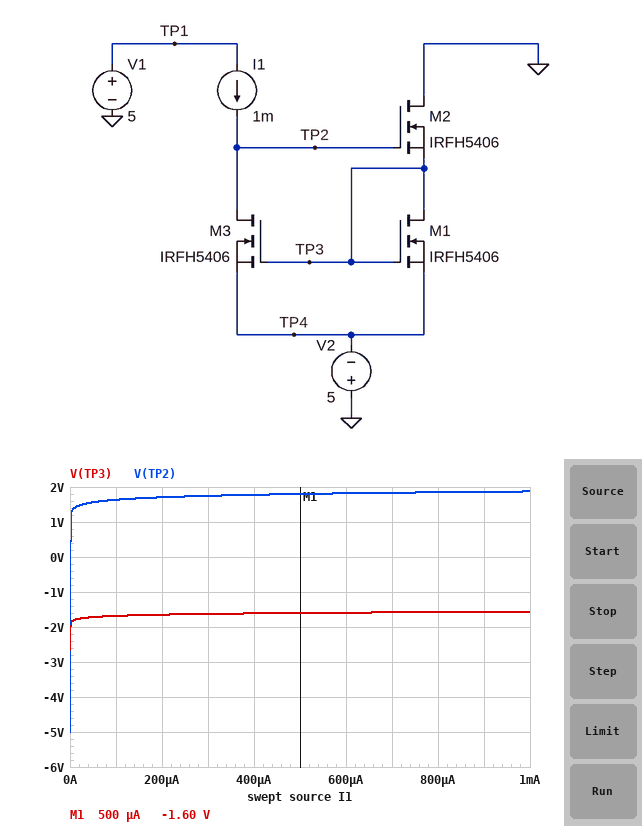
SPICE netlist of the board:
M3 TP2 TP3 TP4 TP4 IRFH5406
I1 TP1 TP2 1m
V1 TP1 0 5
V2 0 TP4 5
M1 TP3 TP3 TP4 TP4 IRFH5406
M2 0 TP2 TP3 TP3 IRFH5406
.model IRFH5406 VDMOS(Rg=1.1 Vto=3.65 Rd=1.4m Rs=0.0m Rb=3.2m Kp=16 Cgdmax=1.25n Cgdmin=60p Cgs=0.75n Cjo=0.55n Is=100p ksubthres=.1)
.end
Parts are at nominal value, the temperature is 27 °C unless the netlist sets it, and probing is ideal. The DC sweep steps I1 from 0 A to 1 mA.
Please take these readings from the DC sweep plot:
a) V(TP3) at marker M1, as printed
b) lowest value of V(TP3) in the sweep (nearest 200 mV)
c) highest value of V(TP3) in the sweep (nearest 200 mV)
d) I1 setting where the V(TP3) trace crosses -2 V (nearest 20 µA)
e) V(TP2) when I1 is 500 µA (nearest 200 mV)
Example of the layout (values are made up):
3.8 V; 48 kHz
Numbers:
-1.60 V; -2.6 V; -1.6 V; 0 A; 1.8 V
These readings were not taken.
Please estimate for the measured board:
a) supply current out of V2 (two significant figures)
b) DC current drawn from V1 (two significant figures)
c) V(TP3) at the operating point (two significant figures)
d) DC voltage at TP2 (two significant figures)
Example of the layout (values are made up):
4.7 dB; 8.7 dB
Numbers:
2.0 mA; 1.0 mA; -1.6 V; 1.9 V
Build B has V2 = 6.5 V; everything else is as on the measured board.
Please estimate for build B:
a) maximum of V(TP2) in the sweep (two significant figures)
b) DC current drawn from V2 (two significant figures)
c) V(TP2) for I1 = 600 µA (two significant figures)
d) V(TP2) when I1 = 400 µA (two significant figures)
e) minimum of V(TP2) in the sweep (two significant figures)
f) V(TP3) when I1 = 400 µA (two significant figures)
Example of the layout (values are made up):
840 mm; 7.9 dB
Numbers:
370 mV; 2.0 mA; 320 mV; 280 mV; -6.5 V; -3.1 V
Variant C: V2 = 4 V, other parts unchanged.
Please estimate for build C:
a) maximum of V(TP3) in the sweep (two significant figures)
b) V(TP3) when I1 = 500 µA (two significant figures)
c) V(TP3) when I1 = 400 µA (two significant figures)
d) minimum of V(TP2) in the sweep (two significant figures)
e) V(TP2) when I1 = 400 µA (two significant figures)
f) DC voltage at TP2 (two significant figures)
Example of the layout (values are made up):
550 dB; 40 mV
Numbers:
-560 mV; -600 mV; -610 mV; -4.0 V; 2.8 V; 2.9 V
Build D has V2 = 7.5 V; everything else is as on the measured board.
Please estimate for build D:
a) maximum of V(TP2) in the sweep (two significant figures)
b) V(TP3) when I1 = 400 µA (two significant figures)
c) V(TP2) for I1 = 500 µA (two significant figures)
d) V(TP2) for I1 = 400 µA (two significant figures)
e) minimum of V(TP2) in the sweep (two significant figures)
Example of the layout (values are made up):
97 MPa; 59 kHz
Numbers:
-630 mV; -4.1 V; -700 mV; -720 mV; -7.5 V
